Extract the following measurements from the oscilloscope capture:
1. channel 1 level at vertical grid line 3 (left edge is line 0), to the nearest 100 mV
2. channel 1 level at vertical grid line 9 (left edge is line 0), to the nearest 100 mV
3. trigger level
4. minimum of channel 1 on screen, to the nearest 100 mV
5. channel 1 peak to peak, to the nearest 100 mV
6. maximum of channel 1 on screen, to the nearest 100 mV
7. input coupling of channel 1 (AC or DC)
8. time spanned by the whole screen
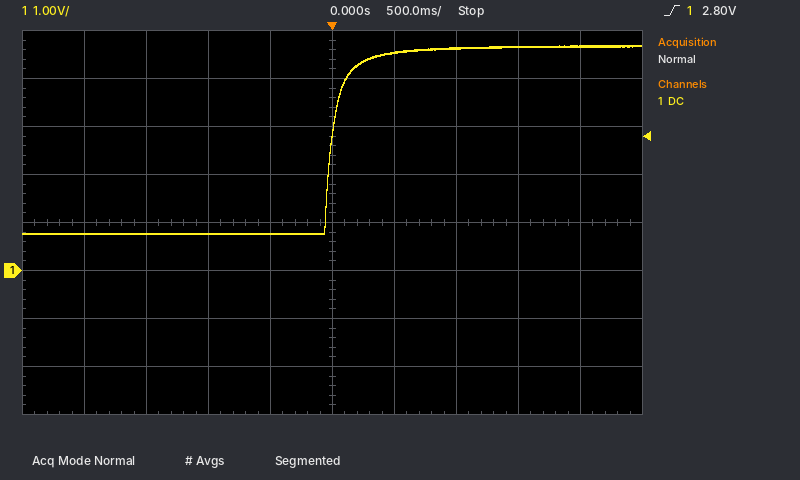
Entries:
800 mV
4.7 V
2.80 V
800 mV
3.9 V
4.7 V
DC
5 s
